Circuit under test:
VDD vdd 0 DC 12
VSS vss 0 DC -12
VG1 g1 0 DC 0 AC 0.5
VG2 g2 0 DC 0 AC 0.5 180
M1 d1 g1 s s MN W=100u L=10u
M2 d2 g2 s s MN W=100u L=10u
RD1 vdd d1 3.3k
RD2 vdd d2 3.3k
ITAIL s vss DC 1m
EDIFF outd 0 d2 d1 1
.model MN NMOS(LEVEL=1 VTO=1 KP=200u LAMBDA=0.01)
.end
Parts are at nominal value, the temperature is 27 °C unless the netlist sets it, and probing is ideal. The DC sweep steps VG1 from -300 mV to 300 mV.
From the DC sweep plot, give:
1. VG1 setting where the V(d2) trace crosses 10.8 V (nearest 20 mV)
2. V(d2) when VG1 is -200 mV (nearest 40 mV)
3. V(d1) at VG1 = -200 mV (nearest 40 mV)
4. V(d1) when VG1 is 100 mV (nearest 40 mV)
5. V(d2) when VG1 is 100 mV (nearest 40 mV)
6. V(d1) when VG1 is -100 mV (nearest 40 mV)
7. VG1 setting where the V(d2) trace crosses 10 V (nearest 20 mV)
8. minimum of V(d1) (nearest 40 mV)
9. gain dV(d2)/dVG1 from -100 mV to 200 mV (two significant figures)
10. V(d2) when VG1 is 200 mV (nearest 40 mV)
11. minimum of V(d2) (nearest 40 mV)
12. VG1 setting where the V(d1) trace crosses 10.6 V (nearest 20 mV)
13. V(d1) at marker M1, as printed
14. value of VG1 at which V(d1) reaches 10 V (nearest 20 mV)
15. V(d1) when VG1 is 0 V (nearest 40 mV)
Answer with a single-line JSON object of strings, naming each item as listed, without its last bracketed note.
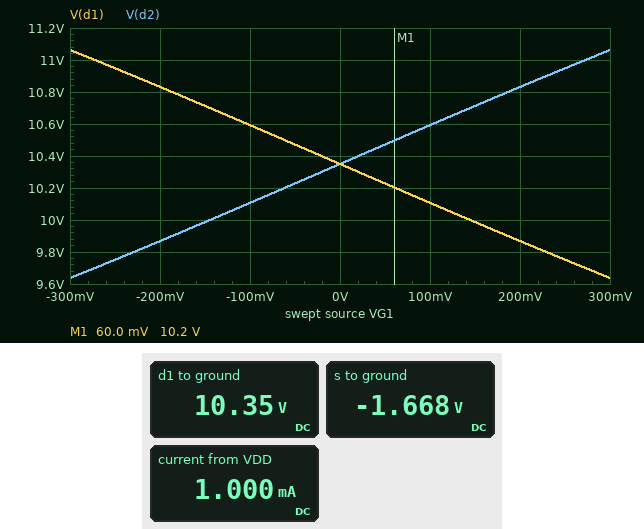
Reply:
{"VG1 setting where the V(d2) trace crosses 10.8 V": "180 mV", "V(d2) when VG1 is -200 mV": "9.88 V", "V(d1) at VG1 = -200 mV": "10.84 V", "V(d1) when VG1 is 100 mV": "10.12 V", "V(d2) when VG1 is 100 mV": "10.60 V", "V(d1) when VG1 is -100 mV": "10.60 V", "VG1 setting where the V(d2) trace crosses 10 V": "-140 mV", "minimum of V(d1)": "9.64 V", "gain dV(d2)/dVG1 from -100 mV to 200 mV": "2.4 V/V", "V(d2) when VG1 is 200 mV": "10.84 V", "minimum of V(d2)": "9.64 V", "VG1 setting where the V(d1) trace crosses 10.6 V": "-100 mV", "V(d1) at marker M1, as printed": "10.2 V", "value of VG1 at which V(d1) reaches 10 V": "140 mV", "V(d1) when VG1 is 0 V": "10.36 V"}
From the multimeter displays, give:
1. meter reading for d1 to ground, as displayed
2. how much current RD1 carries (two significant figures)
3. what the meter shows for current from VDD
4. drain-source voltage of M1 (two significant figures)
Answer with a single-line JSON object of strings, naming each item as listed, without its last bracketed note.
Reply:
{"meter reading for d1 to ground, as displayed": "10.35 V", "how much current RD1 carries": "500 µA", "what the meter shows for current from VDD": "1.000 mA", "drain-source voltage of M1": "12 V"}
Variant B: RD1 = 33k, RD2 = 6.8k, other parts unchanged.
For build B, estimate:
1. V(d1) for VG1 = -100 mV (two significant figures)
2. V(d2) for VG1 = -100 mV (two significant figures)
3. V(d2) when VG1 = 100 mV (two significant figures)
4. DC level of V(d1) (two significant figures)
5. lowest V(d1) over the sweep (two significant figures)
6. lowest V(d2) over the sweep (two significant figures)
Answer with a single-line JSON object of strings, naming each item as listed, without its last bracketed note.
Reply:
{"V(d1) for VG1 = -100 mV": "-1.2 V", "V(d2) for VG1 = -100 mV": "7.9 V", "V(d2) when VG1 = 100 mV": "8.0 V", "DC level of V(d1)": "-1.4 V", "lowest V(d1) over the sweep": "-1.5 V", "lowest V(d2) over the sweep": "7.1 V"}
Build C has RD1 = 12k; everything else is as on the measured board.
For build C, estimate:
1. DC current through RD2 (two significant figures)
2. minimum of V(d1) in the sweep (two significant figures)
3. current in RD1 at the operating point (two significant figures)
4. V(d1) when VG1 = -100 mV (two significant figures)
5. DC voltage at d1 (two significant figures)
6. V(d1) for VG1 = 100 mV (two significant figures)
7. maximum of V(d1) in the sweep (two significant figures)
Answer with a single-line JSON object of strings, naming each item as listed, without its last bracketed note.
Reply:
{"DC current through RD2": "510 µA", "minimum of V(d1) in the sweep": "3.6 V", "current in RD1 at the operating point": "490 µA", "V(d1) when VG1 = -100 mV": "7.0 V", "DC voltage at d1": "6.1 V", "V(d1) for VG1 = 100 mV": "5.3 V", "maximum of V(d1) in the sweep": "8.6 V"}
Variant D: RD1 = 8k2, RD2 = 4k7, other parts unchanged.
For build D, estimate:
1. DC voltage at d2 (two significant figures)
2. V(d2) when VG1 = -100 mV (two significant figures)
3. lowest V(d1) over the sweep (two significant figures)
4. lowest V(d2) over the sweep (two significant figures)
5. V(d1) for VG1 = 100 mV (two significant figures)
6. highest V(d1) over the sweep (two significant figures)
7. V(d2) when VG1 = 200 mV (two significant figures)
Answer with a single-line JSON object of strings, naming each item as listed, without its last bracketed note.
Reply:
{"DC voltage at d2": "9.6 V", "V(d2) when VG1 = -100 mV": "9.3 V", "lowest V(d1) over the sweep": "6.2 V", "lowest V(d2) over the sweep": "8.6 V", "V(d1) for VG1 = 100 mV": "7.3 V", "highest V(d1) over the sweep": "9.7 V", "V(d2) when VG1 = 200 mV": "10 V"}
